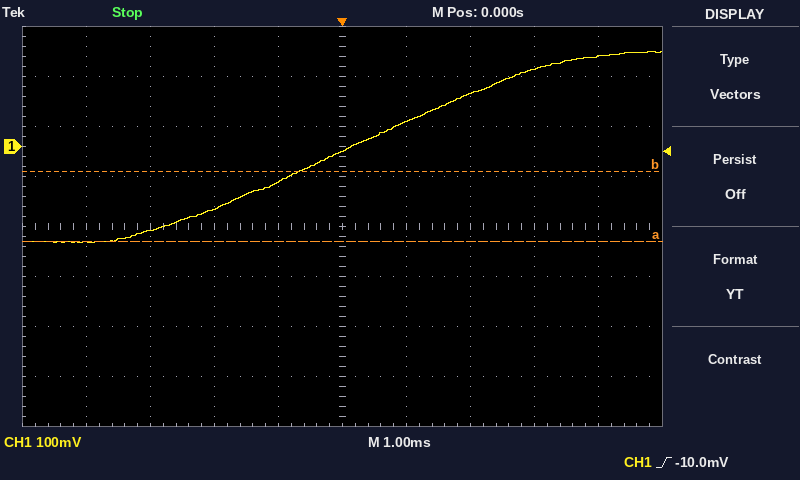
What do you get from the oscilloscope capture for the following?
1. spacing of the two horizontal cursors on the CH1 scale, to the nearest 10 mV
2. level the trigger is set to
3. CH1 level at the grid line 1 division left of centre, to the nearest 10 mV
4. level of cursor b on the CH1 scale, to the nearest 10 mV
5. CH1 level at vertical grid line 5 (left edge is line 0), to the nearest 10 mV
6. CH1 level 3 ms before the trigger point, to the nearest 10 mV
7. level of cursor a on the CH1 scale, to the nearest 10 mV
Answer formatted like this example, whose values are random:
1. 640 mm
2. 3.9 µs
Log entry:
1. 140 mV
2. -10.0 mV
3. -70 mV
4. -50 mV
5. -10 mV
6. -170 mV
7. -190 mV
